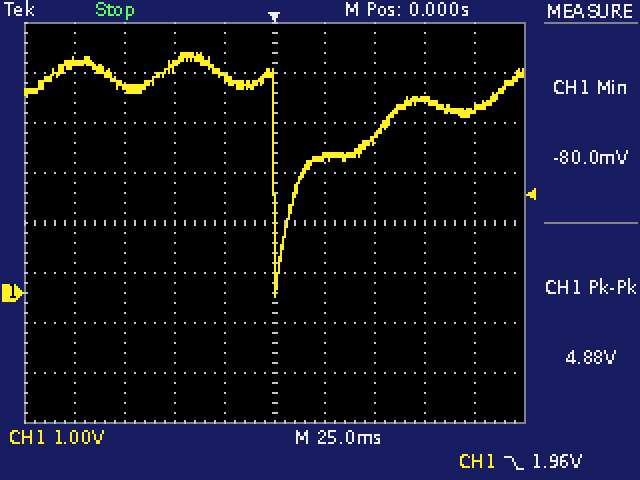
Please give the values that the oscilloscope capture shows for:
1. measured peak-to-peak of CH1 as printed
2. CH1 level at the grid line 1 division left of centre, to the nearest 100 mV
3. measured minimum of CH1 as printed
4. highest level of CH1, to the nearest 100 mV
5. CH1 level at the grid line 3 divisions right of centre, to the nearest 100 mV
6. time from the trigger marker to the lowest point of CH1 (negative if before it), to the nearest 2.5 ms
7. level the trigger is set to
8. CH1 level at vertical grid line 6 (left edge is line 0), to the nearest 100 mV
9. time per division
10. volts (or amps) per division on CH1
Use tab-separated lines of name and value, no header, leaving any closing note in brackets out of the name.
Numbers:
measured peak-to-peak of CH1 as printed	4.88 V
CH1 level at the grid line 1 division left of centre, to the nearest 100 mV	4.3 V
measured minimum of CH1 as printed	-80.0 mV
highest level of CH1, to the nearest 100 mV	4.8 V
CH1 level at the grid line 3 divisions right of centre, to the nearest 100 mV	3.9 V
time from the trigger marker to the lowest point of CH1 (negative if before it), to the nearest 2.5 ms	0.0 ms
level the trigger is set to	1.96 V
CH1 level at vertical grid line 6 (left edge is line 0), to the nearest 100 mV	2.7 V
time per division	25 ms
volts (or amps) per division on CH1	1 V
